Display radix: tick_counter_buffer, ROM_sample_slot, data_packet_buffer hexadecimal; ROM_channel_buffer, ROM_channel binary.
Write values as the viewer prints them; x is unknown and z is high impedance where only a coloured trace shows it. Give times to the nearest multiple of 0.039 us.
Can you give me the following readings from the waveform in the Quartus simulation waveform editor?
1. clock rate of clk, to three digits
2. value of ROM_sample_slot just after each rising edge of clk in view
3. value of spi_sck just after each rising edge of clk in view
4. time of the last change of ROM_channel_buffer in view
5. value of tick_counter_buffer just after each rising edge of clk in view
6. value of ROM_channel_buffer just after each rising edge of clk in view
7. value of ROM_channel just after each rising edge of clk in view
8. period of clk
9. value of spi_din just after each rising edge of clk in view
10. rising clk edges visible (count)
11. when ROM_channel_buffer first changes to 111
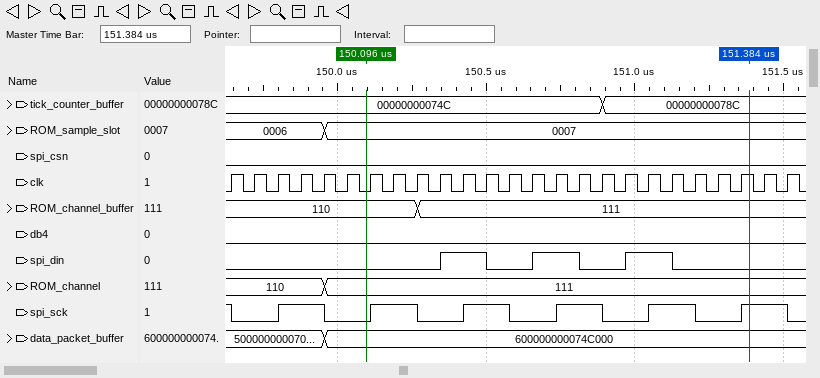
12.8 MHz
0006, 0006, 0006, 0006, 0007, 0007, 0007, 0007, 0007, 0007, 0007, 0007, 0007, 0007, 0007, 0007, 0007, 0007, 0007, 0007, 0007, 0007, 0007, 0007, 0007
0 0 1 1 0 0 1 1 0 0 1 1 0 0 1 1 0 0 1 1 0 0 1 1 0
150.267 us
00000000074C, 00000000074C, 00000000074C, 00000000074C, 00000000074C, 00000000074C, 00000000074C, 00000000074C, 00000000074C, 00000000074C, 00000000074C, 00000000074C, 00000000074C, 00000000074C, 00000000074C, 00000000074C, 00000000078C, 00000000078C, 00000000078C, 00000000078C, 00000000078C, 00000000078C, 00000000078C, 00000000078C, 00000000078C
110, 110, 110, 110, 110, 110, 110, 110, 111, 111, 111, 111, 111, 111, 111, 111, 111, 111, 111, 111, 111, 111, 111, 111, 111
110, 110, 110, 110, 111, 111, 111, 111, 111, 111, 111, 111, 111, 111, 111, 111, 111, 111, 111, 111, 111, 111, 111, 111, 111
0.078 us
0 0 0 0 0 0 0 0 0 1 1 0 0 1 1 0 0 1 1 0 0 0 0 0 0
25
150.267 us
